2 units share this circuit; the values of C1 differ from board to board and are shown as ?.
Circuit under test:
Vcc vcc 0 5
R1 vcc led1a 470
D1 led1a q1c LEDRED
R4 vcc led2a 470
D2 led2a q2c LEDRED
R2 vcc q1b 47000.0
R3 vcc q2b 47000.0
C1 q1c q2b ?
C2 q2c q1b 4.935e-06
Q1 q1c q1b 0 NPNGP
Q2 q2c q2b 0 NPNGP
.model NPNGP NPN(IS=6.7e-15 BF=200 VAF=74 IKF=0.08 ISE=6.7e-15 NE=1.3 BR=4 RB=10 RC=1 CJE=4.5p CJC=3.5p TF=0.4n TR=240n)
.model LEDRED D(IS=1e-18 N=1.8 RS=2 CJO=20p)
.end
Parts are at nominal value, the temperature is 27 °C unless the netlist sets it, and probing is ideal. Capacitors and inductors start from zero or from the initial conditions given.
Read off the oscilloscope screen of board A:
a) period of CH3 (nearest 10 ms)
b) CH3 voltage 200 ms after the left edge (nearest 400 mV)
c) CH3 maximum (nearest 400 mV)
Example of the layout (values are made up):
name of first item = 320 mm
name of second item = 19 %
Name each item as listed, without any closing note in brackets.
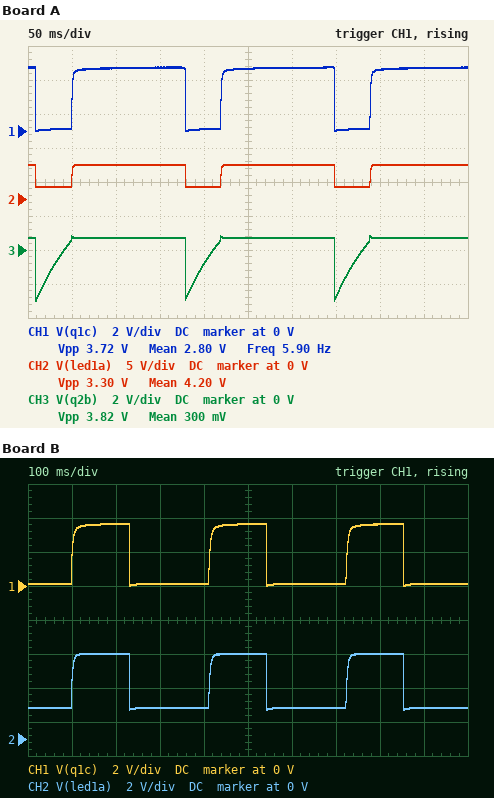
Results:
period of CH3 = 170 ms
CH3 voltage 200 ms after the left edge = -800 mV
CH3 maximum = 800 mV
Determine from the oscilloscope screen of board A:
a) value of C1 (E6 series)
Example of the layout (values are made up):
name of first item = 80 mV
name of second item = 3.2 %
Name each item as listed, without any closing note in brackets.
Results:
value of C1 = 1.5 µF
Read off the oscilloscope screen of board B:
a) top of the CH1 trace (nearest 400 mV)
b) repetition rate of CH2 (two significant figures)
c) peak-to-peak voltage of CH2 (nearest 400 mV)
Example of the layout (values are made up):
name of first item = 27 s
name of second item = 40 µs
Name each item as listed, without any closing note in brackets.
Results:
top of the CH1 trace = 3.6 V
repetition rate of CH2 = 3.2 Hz
peak-to-peak voltage of CH2 = 3.2 V
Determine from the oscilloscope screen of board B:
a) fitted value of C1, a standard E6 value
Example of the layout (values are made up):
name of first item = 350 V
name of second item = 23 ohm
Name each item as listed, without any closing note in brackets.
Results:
fitted value of C1, a standard E6 value = 6.8 µF
